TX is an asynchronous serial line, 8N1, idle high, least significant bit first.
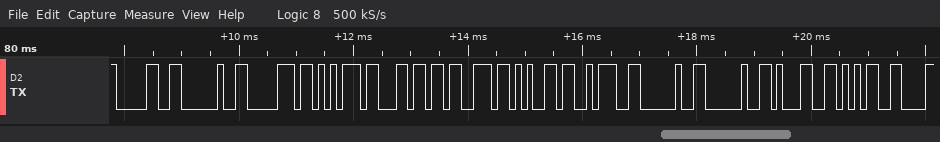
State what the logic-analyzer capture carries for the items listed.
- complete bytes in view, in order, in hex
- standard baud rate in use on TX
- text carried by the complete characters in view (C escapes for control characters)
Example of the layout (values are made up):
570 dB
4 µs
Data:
30 20 70 75 6C 73 65 3A 20 20 31 35
9600 baud
"0 pulse:  15"
